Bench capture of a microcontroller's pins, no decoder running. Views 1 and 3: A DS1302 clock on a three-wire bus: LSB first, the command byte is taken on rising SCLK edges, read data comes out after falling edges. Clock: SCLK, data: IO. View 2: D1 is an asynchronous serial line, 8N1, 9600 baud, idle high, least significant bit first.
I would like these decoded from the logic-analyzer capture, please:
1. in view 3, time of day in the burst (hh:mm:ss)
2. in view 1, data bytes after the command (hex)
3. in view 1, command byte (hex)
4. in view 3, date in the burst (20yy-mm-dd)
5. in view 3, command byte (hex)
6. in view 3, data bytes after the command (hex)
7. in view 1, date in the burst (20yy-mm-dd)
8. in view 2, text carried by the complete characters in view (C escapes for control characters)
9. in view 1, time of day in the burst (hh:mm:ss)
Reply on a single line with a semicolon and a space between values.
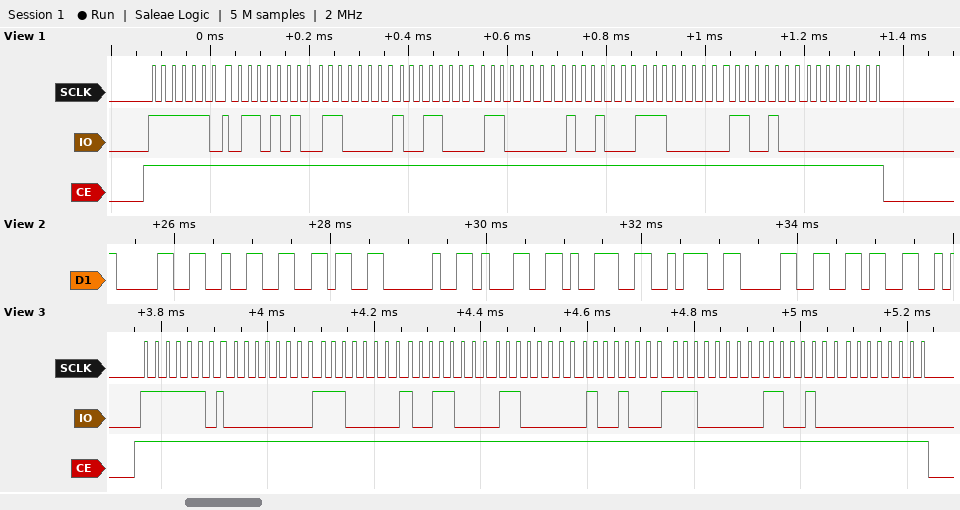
19:07:00; 56 06 19 06 12 07 26 00; 0xBF; 2026-12-06; 0xBF; 00 07 19 06 12 07 26 00; 2026-12-06; "026 19:06"; 19:06:56
